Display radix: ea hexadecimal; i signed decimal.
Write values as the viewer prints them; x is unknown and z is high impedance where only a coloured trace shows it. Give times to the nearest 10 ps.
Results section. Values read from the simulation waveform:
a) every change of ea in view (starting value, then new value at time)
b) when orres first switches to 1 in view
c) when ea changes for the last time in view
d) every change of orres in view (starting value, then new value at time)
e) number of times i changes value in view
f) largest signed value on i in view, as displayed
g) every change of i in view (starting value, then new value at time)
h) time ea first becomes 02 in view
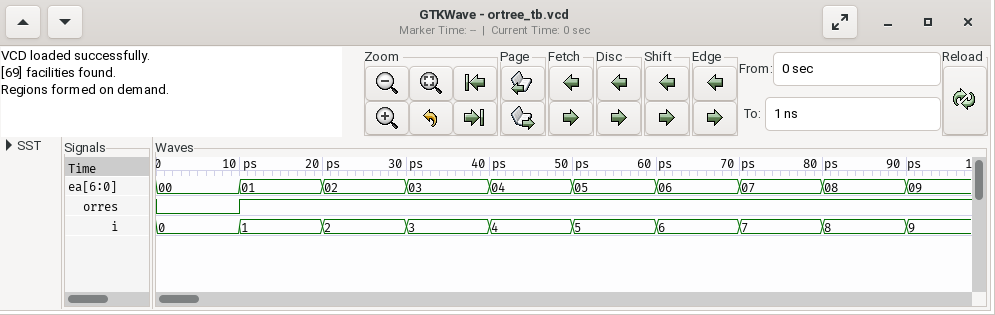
00, 01 at 10 ps, 02 at 20 ps, 03 at 30 ps, 04 at 40 ps, 05 at 50 ps, 06 at 60 ps, 07 at 70 ps, 08 at 80 ps, 09 at 90 ps
10 ps
90 ps
0, 1 at 10 ps
9
9
0, 1 at 10 ps, 2 at 20 ps, 3 at 30 ps, 4 at 40 ps, 5 at 50 ps, 6 at 60 ps, 7 at 70 ps, 8 at 80 ps, 9 at 90 ps
20 ps
